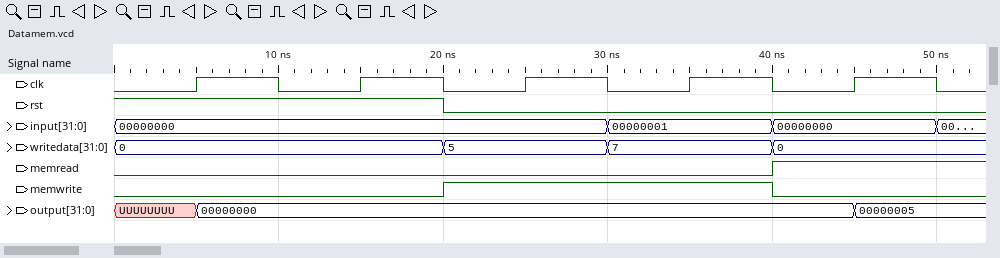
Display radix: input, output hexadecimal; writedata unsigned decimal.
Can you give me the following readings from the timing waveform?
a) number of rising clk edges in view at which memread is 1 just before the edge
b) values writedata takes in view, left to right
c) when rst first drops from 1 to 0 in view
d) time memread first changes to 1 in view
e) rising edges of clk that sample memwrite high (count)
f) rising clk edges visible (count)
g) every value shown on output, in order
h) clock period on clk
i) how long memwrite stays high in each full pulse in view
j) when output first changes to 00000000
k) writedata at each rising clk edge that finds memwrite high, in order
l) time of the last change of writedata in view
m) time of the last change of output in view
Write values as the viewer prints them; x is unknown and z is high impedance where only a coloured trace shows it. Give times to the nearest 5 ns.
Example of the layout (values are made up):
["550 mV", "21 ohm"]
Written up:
["1", "0, 5, 7, 0", "20 ns", "40 ns", "2", "5", "UUUUUUUU, 00000000, 00000005", "10 ns", "20 ns", "5 ns", "5, 7", "40 ns", "45 ns"]
